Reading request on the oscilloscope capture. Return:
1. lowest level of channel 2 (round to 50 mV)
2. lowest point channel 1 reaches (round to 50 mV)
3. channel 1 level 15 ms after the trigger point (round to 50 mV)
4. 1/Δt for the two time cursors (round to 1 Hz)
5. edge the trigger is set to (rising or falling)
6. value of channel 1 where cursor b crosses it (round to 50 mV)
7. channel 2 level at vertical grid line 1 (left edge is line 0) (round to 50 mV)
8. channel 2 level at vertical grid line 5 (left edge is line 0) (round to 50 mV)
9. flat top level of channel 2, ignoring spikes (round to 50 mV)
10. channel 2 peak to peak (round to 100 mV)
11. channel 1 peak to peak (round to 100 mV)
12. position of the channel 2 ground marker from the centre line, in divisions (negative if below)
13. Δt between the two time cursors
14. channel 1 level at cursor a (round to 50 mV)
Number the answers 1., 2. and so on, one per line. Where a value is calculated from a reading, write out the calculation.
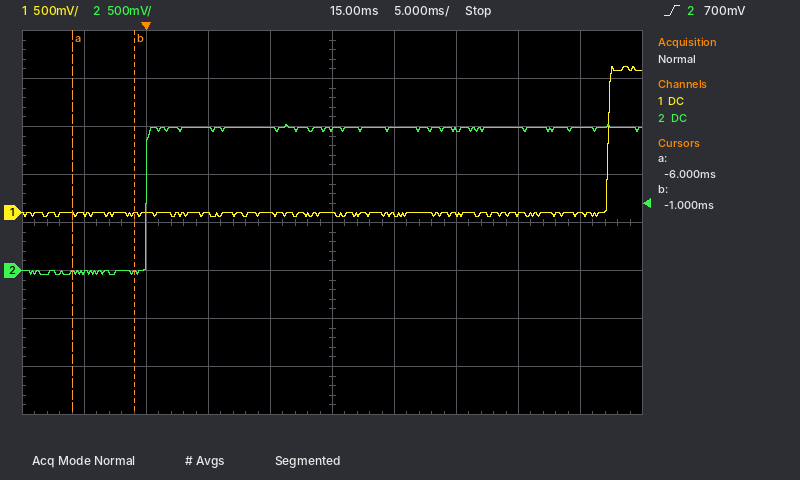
1. -50 mV
2. -50 mV
3. 0 mV
4. 1 / 5.0 ms ≈ 200 Hz
5. rising
6. 0 mV
7. 0 mV
8. 1.45 V
9. 1.50 V
10. 1.60 V
11. 1.60 V
12. -1.0 div
13. -1 ms − (-6 ms) = 5.0 ms
14. 0 mV
